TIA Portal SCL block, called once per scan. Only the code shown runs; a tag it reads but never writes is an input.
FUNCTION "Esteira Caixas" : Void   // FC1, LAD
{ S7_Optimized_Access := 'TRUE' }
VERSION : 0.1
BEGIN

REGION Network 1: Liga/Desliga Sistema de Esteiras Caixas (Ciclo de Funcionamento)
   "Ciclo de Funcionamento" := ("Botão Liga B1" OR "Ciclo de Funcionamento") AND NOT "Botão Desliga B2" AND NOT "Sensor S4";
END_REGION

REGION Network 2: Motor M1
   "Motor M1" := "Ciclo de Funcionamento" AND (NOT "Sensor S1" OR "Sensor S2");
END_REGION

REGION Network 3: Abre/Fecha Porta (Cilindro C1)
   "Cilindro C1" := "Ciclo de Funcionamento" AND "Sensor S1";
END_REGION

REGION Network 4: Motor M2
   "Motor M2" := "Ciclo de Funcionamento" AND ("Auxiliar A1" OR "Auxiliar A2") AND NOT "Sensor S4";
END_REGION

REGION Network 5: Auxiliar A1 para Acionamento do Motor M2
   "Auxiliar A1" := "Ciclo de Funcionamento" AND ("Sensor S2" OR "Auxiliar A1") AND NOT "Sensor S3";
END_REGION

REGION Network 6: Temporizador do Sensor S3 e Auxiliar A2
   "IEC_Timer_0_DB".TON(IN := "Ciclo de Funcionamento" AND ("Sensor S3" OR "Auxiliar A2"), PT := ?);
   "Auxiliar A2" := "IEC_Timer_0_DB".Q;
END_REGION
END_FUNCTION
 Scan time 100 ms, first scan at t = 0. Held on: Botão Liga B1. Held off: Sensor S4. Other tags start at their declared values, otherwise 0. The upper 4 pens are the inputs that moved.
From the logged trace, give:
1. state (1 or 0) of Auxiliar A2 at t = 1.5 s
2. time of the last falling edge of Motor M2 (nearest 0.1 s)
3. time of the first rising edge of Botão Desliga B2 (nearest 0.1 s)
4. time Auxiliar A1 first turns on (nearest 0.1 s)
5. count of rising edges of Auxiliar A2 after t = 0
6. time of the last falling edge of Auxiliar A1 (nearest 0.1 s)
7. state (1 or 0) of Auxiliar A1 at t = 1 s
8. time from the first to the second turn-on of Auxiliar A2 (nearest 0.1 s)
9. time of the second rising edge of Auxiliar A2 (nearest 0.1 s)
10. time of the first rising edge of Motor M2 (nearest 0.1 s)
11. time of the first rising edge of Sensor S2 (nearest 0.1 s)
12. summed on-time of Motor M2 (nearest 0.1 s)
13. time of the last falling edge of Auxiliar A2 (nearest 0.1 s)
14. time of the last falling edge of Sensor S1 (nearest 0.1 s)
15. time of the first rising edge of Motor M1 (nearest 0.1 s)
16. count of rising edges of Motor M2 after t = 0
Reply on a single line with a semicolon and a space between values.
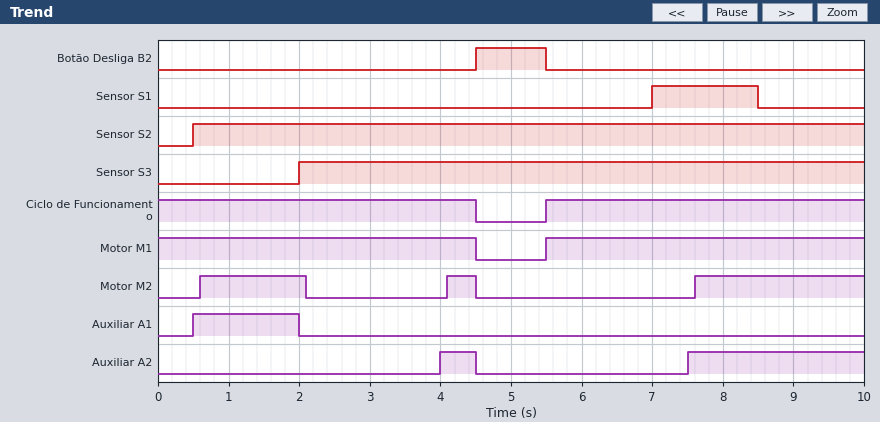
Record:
0; 4.5 s; 4.5 s; 0.5 s; 2; 2.0 s; 1; 3.5 s; 7.5 s; 0.6 s; 0.5 s; 4.3 s; 4.5 s; 8.5 s; 5.5 s; 3
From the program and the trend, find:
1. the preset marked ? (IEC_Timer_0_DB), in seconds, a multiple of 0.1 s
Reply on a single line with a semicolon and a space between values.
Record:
2.0 s
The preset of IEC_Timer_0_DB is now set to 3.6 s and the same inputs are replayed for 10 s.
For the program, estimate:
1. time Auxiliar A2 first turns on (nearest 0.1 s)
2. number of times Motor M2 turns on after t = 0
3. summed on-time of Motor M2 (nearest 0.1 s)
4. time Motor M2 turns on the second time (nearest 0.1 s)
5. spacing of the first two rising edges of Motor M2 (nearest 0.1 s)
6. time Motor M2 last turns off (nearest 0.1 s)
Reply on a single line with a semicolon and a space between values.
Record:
9.1 s; 2; 2.3 s; 9.2 s; 8.6 s; 2.1 s
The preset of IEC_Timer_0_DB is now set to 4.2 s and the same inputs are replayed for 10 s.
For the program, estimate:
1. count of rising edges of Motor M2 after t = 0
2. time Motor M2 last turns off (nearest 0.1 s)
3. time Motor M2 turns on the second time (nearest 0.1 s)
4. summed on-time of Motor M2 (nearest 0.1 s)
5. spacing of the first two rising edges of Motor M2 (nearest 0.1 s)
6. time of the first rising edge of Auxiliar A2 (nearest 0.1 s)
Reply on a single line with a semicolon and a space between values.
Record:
2; 2.1 s; 9.8 s; 1.7 s; 9.2 s; 9.7 s
